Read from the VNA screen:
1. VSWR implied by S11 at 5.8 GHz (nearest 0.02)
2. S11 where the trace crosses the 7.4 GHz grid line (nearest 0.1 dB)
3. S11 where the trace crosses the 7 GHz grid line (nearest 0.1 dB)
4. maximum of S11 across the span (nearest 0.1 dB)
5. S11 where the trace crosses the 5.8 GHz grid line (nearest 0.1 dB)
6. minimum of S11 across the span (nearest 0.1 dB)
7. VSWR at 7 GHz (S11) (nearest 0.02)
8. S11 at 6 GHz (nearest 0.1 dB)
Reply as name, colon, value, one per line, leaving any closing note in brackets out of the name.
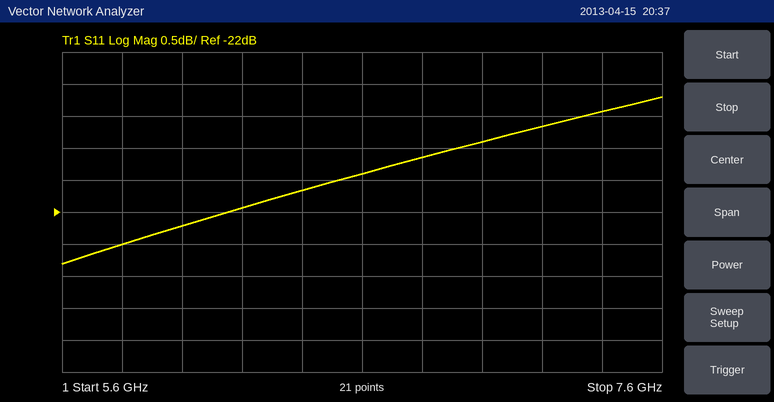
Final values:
VSWR implied by S11 at 5.8 GHz: 1.16
S11 where the trace crosses the 7.4 GHz grid line: -20.4 dB
S11 where the trace crosses the 7 GHz grid line: -20.9 dB
maximum of S11 across the span: -20.2 dB
S11 where the trace crosses the 5.8 GHz grid line: -22.5 dB
minimum of S11 across the span: -22.8 dB
VSWR at 7 GHz (S11): 1.20
S11 at 6 GHz: -22.2 dB
